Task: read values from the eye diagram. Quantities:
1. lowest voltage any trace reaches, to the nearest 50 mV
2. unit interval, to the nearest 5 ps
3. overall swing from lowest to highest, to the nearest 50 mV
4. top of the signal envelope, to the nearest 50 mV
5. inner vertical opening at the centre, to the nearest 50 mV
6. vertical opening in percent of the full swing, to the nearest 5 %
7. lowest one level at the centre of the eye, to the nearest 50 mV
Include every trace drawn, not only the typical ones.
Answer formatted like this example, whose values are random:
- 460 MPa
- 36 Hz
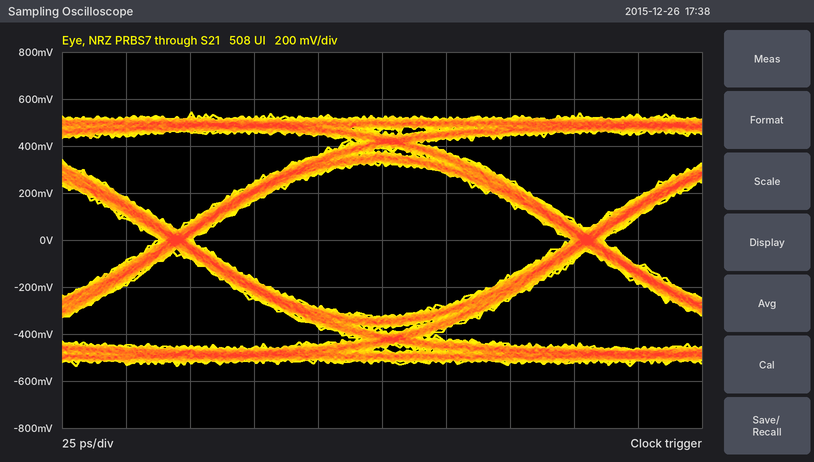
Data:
- -550 mV
- 160 ps
- 1.10 V
- 550 mV
- 650 mV
- 60 %
- 350 mV
